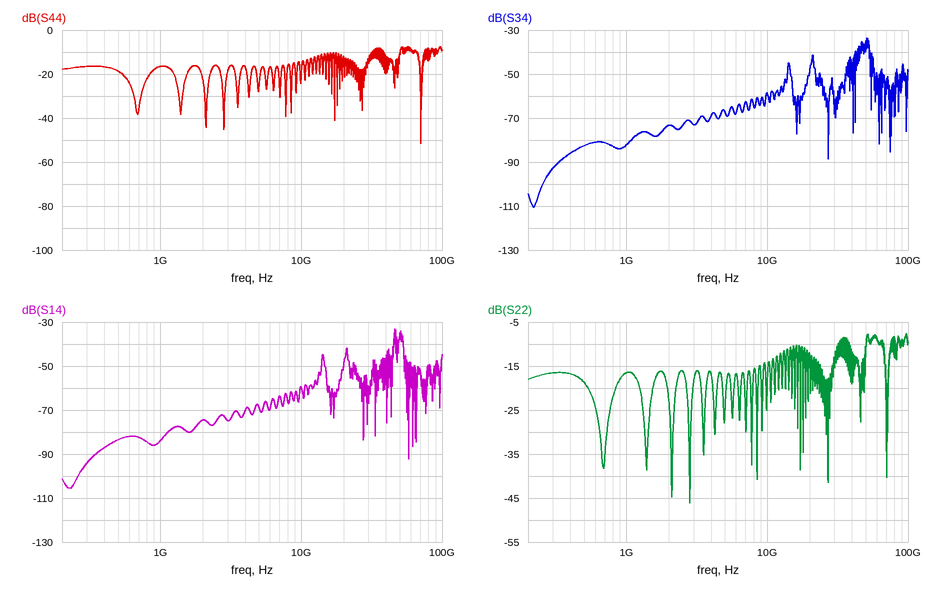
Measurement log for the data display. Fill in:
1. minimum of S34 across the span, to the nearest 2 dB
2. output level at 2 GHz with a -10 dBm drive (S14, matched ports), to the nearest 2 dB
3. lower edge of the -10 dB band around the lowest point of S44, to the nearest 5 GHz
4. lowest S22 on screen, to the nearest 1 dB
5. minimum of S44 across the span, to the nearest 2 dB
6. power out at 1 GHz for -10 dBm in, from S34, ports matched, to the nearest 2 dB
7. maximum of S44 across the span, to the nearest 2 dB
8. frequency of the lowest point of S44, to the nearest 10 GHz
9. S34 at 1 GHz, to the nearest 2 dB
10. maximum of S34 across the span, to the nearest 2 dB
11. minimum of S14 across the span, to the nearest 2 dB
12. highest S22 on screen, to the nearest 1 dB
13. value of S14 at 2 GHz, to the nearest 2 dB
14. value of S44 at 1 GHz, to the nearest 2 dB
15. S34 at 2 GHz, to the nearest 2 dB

-110 dB
-84 dBm
65 GHz
-46 dB
-52 dB
-92 dBm
-8 dB
70 GHz
-82 dB
-34 dB
-106 dB
-8 dB
-74 dB
-16 dB
-74 dB
